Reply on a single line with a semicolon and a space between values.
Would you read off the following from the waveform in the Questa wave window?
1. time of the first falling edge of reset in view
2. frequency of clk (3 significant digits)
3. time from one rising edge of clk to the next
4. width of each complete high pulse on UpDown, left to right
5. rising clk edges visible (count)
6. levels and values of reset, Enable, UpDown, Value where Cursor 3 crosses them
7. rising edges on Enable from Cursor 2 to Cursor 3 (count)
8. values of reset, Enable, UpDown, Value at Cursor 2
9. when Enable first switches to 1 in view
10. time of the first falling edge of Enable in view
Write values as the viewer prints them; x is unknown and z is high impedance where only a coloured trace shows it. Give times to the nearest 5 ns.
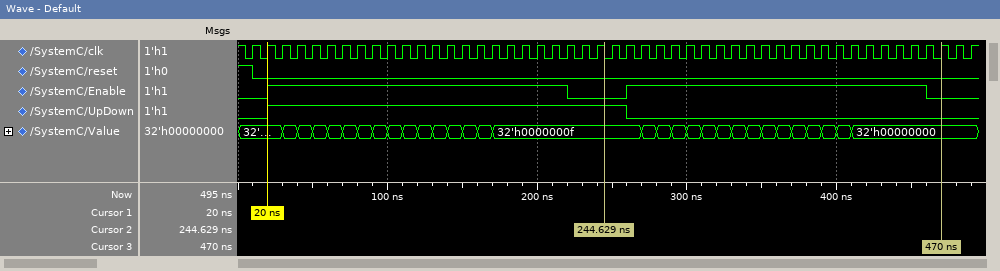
10 ns; 100 MHz; 10 ns; 240 ns; 49; reset=0, Enable=0, UpDown=0, Value=32'h00000000; 1; reset=0, Enable=0, UpDown=1, Value=32'h0000000f; 20 ns; 220 ns
